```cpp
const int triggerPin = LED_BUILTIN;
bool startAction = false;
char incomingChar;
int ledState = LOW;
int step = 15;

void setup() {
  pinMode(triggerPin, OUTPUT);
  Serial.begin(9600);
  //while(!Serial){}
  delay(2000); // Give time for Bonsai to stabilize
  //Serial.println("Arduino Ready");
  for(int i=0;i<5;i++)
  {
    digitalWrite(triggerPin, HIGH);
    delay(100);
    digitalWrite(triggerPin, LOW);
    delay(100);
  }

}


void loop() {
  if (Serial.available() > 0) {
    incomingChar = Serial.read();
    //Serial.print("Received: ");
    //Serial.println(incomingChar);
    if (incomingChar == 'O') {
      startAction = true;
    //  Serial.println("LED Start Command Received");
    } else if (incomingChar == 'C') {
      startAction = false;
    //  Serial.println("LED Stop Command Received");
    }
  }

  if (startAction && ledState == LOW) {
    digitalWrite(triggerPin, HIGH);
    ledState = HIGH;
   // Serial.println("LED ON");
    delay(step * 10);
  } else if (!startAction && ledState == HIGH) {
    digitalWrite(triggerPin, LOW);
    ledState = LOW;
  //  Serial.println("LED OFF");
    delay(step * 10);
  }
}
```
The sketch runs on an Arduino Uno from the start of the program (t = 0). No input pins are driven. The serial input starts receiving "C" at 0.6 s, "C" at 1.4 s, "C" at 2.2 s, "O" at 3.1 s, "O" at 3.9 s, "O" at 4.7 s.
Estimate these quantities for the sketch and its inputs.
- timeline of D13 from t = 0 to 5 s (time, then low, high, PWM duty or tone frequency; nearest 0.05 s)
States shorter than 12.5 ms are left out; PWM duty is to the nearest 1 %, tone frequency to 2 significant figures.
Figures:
0 s low; 2 s high; 2.1 s low; 2.2 s high; 2.3 s low; 2.4 s high; 2.5 s low; 2.6 s high; 2.7 s low; 2.8 s high; 2.9 s low; 3.1 s high
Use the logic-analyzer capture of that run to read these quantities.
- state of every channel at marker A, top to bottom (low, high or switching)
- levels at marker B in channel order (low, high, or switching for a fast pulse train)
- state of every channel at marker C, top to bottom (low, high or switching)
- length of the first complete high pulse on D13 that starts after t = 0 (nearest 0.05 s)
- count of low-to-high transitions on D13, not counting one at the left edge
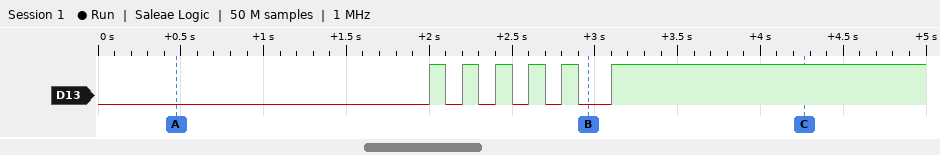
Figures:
D13 low
D13 low
D13 high
0.10 s
6
